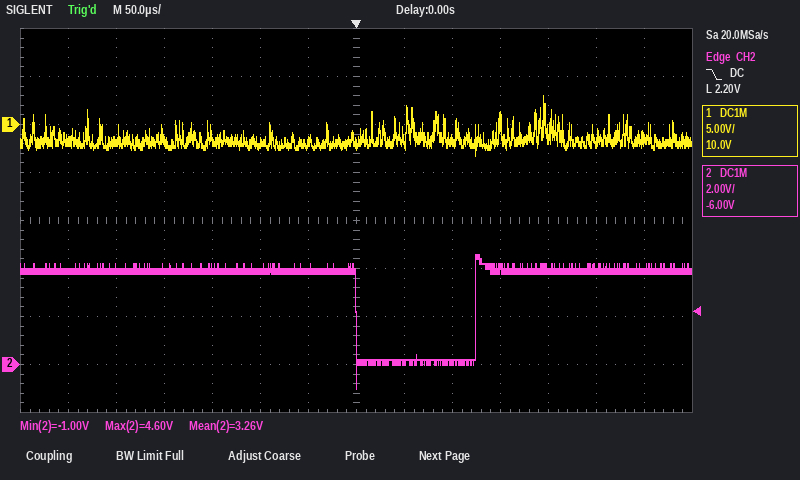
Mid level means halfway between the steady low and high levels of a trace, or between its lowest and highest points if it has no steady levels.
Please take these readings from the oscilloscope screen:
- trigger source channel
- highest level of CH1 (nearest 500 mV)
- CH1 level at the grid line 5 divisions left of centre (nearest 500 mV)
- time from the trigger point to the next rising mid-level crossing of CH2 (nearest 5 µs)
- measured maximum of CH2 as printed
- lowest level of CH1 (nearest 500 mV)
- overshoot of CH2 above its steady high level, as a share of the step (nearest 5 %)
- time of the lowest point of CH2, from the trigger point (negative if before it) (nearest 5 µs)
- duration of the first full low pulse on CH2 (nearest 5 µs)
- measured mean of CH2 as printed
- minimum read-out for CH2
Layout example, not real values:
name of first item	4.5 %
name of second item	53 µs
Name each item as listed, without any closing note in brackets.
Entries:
trigger source channel	CH2
highest level of CH1	3.0 V
CH1 level at the grid line 5 divisions left of centre	-1.5 V
time from the trigger point to the next rising mid-level crossing of CH2	125 µs
measured maximum of CH2 as printed	4.60 V
lowest level of CH1	-3.0 V
overshoot of CH2 above its steady high level, as a share of the step	20 %
time of the lowest point of CH2, from the trigger point (negative if before it)	0 µs
duration of the first full low pulse on CH2	125 µs
measured mean of CH2 as printed	3.26 V
minimum read-out for CH2	-1.00 V
